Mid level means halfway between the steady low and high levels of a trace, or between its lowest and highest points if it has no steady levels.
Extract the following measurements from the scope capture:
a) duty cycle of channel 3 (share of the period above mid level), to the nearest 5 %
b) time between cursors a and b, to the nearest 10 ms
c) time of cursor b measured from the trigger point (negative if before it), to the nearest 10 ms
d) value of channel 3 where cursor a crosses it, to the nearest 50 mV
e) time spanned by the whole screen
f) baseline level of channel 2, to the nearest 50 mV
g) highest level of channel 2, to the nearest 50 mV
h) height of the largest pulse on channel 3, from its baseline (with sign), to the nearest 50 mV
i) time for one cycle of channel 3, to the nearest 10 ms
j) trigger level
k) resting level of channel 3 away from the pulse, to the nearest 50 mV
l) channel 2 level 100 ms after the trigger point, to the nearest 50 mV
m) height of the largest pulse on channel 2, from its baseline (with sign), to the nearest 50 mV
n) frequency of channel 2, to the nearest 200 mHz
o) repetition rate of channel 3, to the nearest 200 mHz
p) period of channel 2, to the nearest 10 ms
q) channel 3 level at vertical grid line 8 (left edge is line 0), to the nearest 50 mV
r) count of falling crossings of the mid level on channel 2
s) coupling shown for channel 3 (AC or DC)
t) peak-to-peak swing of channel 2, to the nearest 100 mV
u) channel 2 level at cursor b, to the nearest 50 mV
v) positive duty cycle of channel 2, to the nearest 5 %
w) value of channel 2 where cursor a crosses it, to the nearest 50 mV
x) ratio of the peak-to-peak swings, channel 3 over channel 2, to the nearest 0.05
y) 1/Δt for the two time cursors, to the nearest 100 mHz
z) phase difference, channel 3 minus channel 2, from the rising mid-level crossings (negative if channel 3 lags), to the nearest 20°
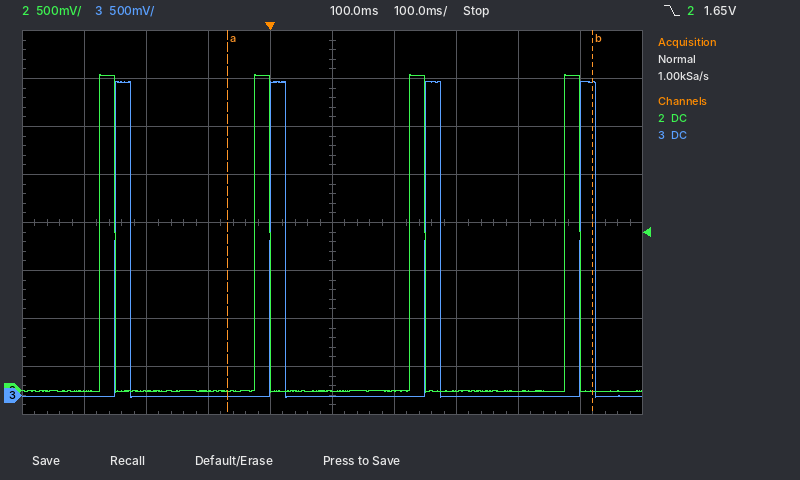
10 %
590 ms
+520 ms
0 mV
1 s
0 mV
3.30 V
+3.30 V
250 ms
1.65 V
0 mV
0 mV
+3.30 V
4.0 Hz
4.0 Hz
250 ms
0 mV
4
DC
3.30 V
0 mV
10 %
0 mV
1.00
1.7 Hz
-40°
